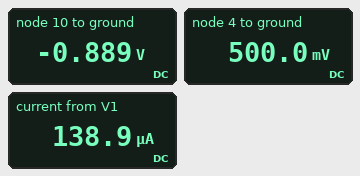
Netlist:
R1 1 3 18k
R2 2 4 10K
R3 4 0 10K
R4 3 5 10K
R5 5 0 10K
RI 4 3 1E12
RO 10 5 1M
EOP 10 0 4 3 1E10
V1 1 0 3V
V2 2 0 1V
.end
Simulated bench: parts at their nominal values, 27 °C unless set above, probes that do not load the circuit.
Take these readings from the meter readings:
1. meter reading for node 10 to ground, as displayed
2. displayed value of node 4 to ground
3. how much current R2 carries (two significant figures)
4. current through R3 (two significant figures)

-0.889 V
500.0 mV
50 µA
50 µA
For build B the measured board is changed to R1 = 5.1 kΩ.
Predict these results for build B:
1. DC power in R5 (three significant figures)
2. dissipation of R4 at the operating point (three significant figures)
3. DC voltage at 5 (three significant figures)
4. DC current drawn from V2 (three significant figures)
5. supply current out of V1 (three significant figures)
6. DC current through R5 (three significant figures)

1.94 mW
2.40 mW
-4.40 V
50.0 µA
490 µA
440 µA
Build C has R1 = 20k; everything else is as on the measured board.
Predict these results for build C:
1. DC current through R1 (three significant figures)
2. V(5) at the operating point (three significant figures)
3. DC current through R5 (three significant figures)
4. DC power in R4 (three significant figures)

125 µA
-750 mV
75.0 µA
156 µW
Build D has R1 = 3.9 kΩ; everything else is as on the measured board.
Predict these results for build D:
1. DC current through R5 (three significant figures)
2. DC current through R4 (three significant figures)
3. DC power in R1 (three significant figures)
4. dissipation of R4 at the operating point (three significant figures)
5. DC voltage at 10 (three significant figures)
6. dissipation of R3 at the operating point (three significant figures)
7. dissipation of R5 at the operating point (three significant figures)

591 µA
641 µA
1.60 mW
4.11 mW
-5.91 V
25.0 µW
3.49 mW
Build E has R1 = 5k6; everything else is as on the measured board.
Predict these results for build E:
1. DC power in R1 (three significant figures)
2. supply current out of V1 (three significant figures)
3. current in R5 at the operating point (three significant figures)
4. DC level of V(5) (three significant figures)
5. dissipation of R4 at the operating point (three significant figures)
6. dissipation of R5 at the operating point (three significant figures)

1.12 mW
446 µA
396 µA
-3.96 V
1.99 mW
1.57 mW
